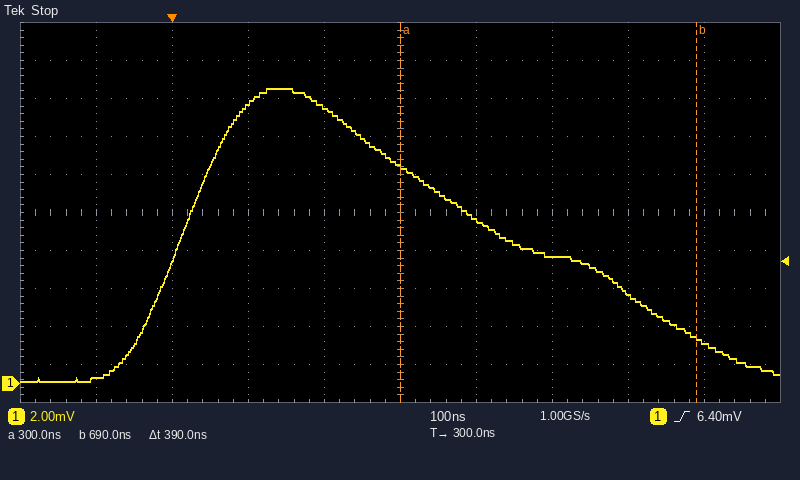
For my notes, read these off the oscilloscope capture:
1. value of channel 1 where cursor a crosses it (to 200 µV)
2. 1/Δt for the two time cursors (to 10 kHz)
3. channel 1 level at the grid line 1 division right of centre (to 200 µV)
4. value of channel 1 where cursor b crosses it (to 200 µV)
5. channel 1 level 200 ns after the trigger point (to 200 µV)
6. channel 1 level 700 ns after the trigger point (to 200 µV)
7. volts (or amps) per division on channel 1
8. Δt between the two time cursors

11.4 mV
2.56 MHz
8.6 mV
2.4 mV
14.6 mV
2.2 mV
2 mV
390 ns
